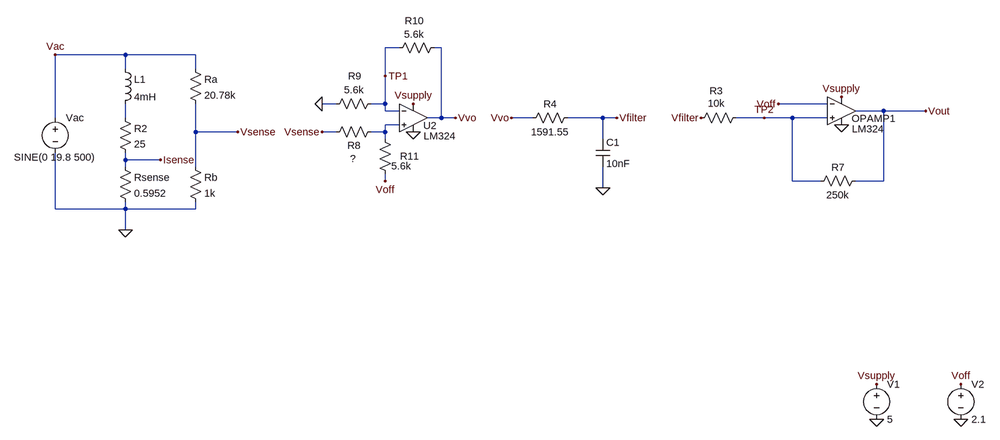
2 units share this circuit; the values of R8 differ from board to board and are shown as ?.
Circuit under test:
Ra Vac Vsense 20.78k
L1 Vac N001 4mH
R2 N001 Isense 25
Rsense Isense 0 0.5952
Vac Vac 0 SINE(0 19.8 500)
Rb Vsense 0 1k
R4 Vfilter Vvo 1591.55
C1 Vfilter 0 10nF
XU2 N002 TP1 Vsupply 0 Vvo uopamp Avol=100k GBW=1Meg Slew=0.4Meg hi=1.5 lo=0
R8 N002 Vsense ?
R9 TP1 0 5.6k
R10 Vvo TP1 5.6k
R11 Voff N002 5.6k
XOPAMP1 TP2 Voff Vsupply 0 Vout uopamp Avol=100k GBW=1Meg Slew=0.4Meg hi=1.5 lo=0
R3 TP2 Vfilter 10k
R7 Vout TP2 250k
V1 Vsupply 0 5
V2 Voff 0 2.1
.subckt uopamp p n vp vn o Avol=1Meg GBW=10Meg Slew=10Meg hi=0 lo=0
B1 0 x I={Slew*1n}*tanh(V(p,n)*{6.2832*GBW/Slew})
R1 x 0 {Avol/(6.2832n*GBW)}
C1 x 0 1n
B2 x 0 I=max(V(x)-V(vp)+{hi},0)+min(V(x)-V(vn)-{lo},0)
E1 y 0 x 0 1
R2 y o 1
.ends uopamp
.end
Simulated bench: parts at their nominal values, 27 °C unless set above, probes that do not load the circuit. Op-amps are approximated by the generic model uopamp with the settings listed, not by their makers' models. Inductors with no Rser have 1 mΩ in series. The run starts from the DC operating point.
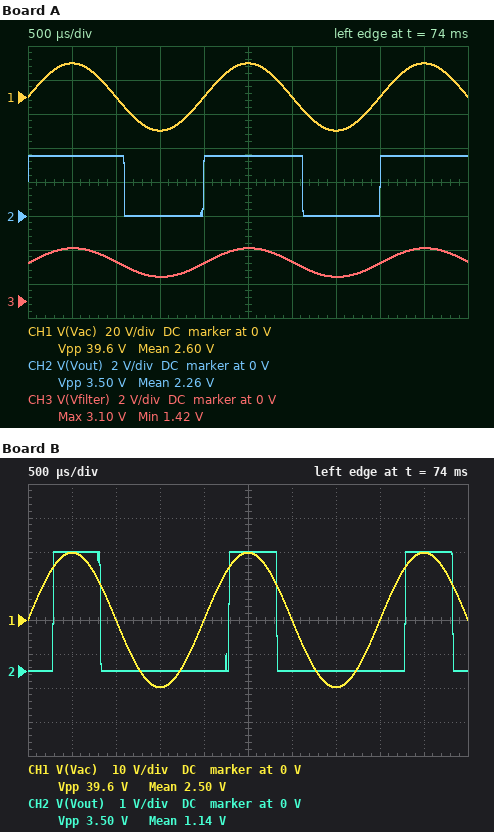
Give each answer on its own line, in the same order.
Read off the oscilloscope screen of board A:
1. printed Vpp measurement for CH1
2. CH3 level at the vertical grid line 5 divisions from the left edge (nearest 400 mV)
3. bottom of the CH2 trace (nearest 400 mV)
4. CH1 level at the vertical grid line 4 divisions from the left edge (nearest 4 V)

39.6 V
3.2 V
0 V
0 V
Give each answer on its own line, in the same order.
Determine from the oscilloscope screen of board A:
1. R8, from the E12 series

5.6 kΩ
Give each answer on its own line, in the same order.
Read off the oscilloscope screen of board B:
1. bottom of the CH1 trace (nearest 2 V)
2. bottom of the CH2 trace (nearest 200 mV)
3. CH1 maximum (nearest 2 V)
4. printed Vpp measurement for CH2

-20 V
0 V
20 V
3.50 V
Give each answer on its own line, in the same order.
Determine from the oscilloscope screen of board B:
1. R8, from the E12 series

1.5 kΩ
